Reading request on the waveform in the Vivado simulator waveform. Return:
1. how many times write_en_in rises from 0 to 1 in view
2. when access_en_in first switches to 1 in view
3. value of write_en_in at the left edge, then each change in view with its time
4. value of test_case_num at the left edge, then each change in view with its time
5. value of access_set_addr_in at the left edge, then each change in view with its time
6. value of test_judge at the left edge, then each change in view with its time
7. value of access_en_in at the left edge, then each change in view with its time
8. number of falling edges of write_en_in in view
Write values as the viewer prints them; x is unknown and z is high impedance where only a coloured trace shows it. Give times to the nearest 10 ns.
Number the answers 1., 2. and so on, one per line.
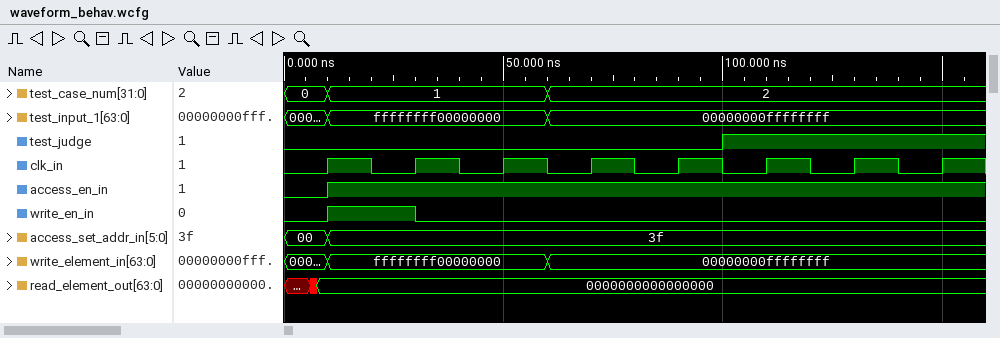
1. 1
2. 10 ns
3. 0, 1 at 10 ns, 0 at 30 ns
4. 0, 1 at 10 ns, 2 at 60 ns
5. 00, 3f at 10 ns
6. 0, 1 at 100 ns
7. 0, 1 at 10 ns
8. 1
